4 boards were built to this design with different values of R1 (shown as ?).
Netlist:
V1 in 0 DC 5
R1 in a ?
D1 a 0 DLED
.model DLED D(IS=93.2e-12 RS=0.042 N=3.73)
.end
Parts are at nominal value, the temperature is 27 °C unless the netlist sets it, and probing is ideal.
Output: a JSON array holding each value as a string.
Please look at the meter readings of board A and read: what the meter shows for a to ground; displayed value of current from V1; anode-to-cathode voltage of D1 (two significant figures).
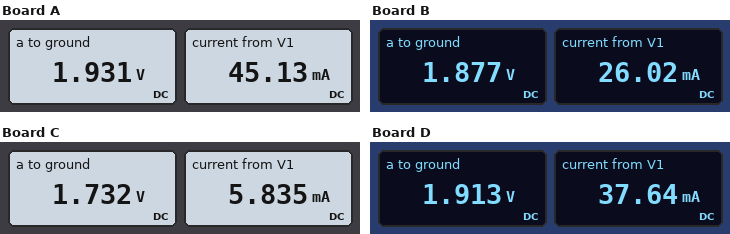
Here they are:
["1.931 V", "45.13 mA", "1.9 V"]
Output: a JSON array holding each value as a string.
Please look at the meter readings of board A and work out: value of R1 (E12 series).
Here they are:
["68 Ω"]
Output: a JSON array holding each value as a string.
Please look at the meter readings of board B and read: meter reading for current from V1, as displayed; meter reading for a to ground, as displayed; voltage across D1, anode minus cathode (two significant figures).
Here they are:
["26.02 mA", "1.877 V", "1.9 V"]
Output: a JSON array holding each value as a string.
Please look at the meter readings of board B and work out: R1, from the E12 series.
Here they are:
["120 Ω"]
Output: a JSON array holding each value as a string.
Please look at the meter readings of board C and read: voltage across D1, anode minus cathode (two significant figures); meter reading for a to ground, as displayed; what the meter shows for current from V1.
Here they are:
["1.7 V", "1.732 V", "5.835 mA"]
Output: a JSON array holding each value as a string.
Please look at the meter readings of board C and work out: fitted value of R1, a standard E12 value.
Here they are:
["560 Ω"]
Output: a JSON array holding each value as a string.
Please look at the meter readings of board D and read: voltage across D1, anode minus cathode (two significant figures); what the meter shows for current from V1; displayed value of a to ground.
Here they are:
["1.9 V", "37.64 mA", "1.913 V"]
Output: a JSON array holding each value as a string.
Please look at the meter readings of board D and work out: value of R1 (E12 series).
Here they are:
["82 Ω"]
